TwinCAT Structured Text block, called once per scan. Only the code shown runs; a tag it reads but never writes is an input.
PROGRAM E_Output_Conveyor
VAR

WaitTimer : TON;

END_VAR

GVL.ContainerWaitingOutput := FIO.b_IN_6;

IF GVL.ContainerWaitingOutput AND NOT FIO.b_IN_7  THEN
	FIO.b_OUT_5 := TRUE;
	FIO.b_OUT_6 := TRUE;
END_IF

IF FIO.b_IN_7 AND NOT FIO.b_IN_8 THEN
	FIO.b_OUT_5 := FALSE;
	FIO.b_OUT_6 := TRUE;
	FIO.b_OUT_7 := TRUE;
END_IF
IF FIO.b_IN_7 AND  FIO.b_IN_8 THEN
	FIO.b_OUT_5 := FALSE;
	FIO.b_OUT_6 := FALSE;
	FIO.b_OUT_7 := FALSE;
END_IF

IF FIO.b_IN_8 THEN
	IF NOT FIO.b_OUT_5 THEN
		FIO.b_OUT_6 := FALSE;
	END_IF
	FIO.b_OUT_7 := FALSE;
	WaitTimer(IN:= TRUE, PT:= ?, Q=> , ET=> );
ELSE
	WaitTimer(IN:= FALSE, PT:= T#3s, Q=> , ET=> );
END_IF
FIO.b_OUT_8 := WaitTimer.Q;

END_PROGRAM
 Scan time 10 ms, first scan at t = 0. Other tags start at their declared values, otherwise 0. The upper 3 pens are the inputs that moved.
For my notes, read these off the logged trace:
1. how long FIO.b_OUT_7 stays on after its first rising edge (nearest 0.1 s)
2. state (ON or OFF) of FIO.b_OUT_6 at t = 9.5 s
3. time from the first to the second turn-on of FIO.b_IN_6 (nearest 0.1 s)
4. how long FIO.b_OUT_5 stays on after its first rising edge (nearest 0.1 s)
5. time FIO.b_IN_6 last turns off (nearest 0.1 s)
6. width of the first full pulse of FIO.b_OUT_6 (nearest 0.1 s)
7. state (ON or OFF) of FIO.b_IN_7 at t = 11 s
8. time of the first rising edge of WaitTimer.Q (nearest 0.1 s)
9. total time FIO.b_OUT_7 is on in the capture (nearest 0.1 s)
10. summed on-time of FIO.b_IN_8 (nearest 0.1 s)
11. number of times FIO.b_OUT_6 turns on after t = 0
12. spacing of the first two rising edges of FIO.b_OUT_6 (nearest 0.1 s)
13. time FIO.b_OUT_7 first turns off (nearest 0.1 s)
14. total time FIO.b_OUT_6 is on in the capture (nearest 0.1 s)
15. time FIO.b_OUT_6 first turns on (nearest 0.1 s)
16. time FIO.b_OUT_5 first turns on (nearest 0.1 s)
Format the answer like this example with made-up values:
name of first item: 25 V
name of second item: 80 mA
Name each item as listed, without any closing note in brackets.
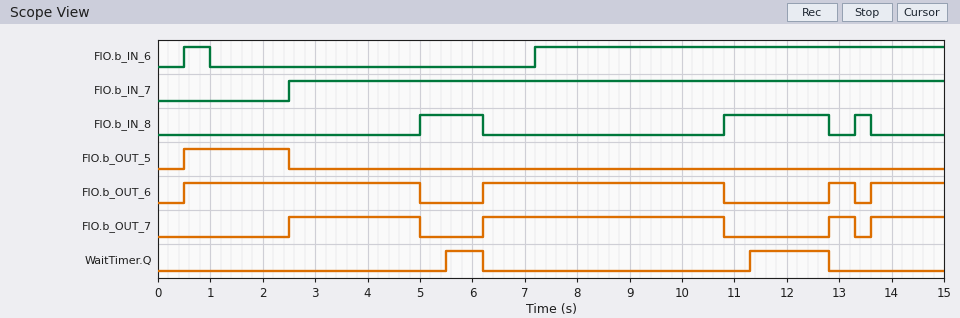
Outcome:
how long FIO.b_OUT_7 stays on after its first rising edge: 2.5 s
state (ON or OFF) of FIO.b_OUT_6 at t = 9.5 s: ON
time from the first to the second turn-on of FIO.b_IN_6: 6.7 s
how long FIO.b_OUT_5 stays on after its first rising edge: 2.0 s
time FIO.b_IN_6 last turns off: 1.0 s
width of the first full pulse of FIO.b_OUT_6: 4.5 s
state (ON or OFF) of FIO.b_IN_7 at t = 11 s: ON
time of the first rising edge of WaitTimer.Q: 5.5 s
total time FIO.b_OUT_7 is on in the capture: 9.0 s
summed on-time of FIO.b_IN_8: 3.5 s
number of times FIO.b_OUT_6 turns on after t = 0: 4
spacing of the first two rising edges of FIO.b_OUT_6: 5.7 s
time FIO.b_OUT_7 first turns off: 5.0 s
total time FIO.b_OUT_6 is on in the capture: 11.0 s
time FIO.b_OUT_6 first turns on: 0.5 s
time FIO.b_OUT_5 first turns on: 0.5 s
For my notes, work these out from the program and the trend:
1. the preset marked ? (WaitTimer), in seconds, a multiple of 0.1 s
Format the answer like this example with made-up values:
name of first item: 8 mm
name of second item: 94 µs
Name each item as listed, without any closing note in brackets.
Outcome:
the preset marked ? (WaitTimer), in seconds, a multiple of 0.1 s: 0.5 s
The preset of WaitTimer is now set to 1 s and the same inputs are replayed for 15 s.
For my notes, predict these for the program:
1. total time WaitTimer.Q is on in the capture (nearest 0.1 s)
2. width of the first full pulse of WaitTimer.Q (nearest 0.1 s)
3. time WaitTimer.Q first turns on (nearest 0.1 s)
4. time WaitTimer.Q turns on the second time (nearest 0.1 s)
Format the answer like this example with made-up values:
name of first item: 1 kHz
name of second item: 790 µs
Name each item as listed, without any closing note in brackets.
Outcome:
total time WaitTimer.Q is on in the capture: 1.2 s
width of the first full pulse of WaitTimer.Q: 0.2 s
time WaitTimer.Q first turns on: 6.0 s
time WaitTimer.Q turns on the second time: 11.8 s
